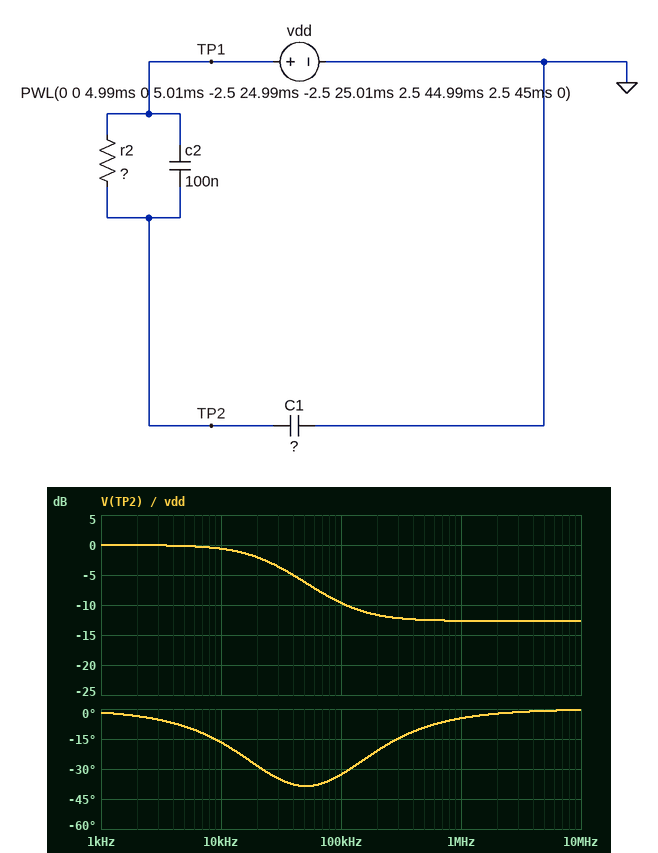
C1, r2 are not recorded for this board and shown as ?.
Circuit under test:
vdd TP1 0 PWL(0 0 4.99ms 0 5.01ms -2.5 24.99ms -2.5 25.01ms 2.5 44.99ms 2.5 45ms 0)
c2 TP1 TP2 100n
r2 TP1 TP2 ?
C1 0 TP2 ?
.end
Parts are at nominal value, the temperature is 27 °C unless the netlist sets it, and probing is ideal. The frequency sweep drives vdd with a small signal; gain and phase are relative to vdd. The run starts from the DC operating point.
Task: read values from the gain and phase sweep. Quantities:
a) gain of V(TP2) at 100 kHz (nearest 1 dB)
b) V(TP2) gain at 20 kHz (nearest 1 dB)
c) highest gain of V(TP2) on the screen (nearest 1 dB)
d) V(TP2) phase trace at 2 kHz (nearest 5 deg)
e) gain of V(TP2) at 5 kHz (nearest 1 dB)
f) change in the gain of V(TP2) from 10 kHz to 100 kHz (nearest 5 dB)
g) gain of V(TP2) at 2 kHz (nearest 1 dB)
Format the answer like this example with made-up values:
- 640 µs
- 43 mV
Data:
- -10 dB
- -2 dB
- 0 dB
- -5 deg
- 0 dB
- -10 dB
- 0 dB
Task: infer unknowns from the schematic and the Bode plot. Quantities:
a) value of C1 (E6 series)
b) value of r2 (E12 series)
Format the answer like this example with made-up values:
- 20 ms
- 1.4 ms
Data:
- 330 nF
- 15 Ω
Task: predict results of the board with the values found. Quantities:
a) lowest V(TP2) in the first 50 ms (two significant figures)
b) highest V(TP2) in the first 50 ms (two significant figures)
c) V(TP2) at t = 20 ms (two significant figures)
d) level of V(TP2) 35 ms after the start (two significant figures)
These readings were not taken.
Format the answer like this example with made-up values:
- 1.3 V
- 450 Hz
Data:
- -2.5 V
- 2.5 V
- -2.5 V
- 2.5 V
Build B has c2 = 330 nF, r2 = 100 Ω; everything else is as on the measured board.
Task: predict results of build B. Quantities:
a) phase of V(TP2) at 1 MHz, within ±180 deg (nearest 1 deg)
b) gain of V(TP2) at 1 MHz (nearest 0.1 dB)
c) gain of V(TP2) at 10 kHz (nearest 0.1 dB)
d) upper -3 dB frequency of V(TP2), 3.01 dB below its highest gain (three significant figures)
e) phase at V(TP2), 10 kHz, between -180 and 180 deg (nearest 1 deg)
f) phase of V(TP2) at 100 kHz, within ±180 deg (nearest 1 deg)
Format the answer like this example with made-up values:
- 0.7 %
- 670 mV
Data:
- 0 deg
- -6.0 dB
- -5.4 dB
- 3.41 kHz
- -12 deg
- -1 deg
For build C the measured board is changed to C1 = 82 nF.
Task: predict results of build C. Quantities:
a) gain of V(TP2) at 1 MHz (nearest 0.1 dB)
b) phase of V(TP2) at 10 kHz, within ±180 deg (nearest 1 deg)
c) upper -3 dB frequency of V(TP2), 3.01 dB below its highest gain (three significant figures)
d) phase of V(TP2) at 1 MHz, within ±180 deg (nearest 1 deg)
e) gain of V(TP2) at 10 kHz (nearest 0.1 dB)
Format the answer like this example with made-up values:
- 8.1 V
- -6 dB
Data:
- -5.2 dB
- -4 deg
- 92.6 kHz
- -3 deg
- -0.1 dB
